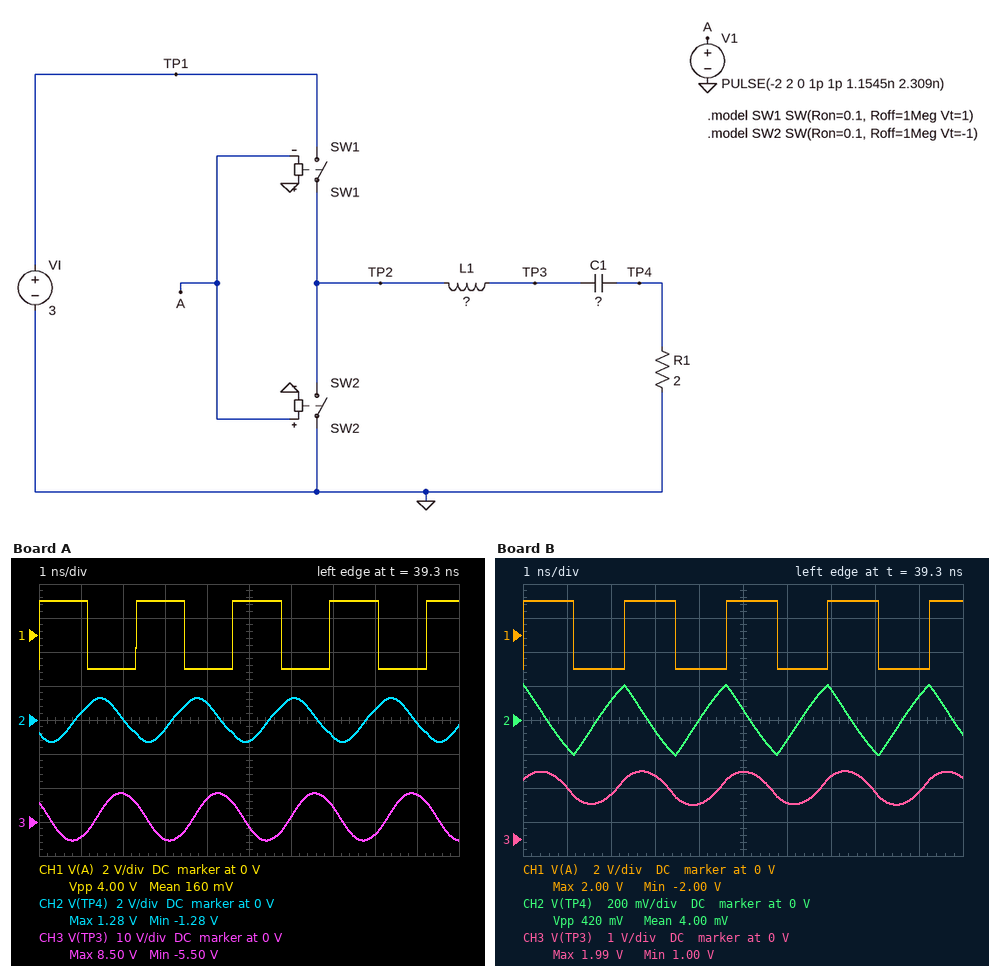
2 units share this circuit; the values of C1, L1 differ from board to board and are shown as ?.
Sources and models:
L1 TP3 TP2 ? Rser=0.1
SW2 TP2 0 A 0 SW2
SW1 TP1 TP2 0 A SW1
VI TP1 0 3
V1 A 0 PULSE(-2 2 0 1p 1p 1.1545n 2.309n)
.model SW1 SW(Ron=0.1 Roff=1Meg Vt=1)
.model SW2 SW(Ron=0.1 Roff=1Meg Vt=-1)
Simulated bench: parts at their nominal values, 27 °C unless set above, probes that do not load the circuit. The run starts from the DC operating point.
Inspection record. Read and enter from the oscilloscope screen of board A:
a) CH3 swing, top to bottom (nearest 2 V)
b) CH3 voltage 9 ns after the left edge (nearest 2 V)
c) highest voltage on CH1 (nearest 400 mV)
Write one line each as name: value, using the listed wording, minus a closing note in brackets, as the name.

CH3 swing, top to bottom: 14 V
CH3 voltage 9 ns after the left edge: 8 V
highest voltage on CH1: 2.0 V
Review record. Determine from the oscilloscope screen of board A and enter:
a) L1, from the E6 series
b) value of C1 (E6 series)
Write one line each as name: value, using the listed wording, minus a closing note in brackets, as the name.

L1, from the E6 series: 3.3 nH
value of C1: 33 pF
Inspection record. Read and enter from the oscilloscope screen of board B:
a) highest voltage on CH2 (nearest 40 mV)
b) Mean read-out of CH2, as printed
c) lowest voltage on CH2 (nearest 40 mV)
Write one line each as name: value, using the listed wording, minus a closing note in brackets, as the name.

highest voltage on CH2: 200 mV
Mean read-out of CH2, as printed: 4.00 mV
lowest voltage on CH2: -200 mV
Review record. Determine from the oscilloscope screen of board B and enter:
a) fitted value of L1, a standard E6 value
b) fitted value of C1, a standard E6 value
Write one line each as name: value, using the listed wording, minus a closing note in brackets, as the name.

fitted value of L1, a standard E6 value: 10 nH
fitted value of C1, a standard E6 value: 68 pF
